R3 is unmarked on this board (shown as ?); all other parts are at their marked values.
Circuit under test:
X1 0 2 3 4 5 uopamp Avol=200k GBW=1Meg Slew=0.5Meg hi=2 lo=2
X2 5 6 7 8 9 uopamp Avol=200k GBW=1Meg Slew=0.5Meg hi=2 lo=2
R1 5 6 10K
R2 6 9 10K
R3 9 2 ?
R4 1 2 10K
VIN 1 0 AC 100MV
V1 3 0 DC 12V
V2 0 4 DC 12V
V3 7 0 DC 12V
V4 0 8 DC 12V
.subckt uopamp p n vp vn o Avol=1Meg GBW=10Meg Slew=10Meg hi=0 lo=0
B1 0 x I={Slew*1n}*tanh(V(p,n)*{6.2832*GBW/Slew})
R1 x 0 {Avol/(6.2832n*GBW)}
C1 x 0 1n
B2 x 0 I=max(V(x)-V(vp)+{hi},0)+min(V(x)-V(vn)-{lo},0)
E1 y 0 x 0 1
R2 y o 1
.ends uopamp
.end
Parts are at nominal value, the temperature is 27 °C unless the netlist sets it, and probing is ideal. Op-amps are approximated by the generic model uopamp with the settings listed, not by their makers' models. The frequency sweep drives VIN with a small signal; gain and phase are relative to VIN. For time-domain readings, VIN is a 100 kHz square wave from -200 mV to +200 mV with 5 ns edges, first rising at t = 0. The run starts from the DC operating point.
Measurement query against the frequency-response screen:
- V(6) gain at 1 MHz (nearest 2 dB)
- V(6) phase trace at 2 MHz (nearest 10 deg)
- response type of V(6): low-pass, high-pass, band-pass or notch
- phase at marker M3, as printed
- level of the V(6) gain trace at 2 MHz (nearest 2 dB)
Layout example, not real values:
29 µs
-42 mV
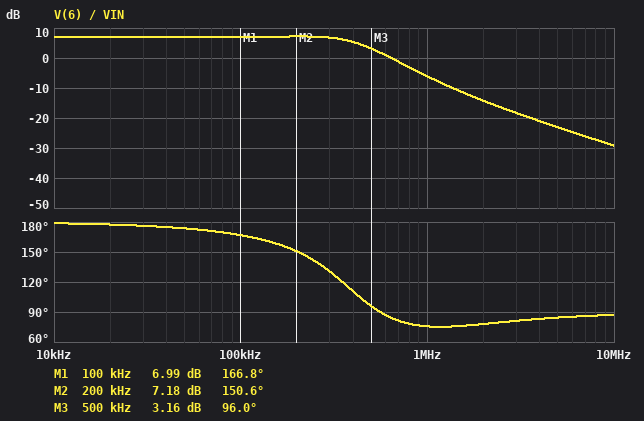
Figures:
-6 dB
80 deg
low-pass
96.0 deg
-14 dB
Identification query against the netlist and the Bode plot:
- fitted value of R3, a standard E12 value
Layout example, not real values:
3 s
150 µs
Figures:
22 kΩ
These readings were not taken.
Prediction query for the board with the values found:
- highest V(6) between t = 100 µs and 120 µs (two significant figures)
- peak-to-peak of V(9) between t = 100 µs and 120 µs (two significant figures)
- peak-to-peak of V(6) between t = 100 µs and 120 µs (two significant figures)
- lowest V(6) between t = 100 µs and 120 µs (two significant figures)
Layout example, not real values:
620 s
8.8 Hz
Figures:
500 mV
990 mV
1.0 V
-500 mV
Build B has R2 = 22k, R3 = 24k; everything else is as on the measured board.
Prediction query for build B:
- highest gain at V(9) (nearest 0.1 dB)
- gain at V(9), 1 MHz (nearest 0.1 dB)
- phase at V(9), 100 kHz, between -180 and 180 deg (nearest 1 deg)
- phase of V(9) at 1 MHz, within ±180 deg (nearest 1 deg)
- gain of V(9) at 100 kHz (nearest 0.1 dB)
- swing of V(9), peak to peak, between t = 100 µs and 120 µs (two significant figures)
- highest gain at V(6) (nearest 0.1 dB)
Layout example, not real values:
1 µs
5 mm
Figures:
8.7 dB
-12.8 dB
159 deg
19 deg
8.0 dB
1.2 V
9.6 dB
